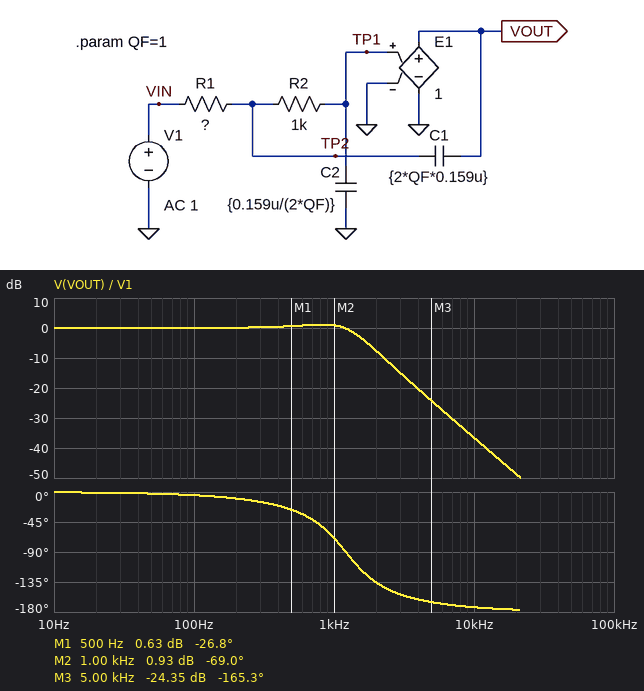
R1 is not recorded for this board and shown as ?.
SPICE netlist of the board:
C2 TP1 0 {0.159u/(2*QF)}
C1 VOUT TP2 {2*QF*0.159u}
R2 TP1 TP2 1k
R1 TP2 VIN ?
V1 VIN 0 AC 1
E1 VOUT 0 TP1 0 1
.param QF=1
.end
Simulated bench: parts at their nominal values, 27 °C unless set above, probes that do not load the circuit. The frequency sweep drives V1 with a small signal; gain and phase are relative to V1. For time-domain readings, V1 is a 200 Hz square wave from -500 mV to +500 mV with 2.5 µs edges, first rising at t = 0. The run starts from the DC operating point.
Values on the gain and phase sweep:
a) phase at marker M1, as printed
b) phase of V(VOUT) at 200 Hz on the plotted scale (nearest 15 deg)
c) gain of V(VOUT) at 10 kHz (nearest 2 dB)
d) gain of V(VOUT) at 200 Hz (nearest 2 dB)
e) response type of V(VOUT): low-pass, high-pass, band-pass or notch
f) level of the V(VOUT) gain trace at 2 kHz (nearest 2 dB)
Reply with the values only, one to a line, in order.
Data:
-26.8 deg
-15 deg
-36 dB
0 dB
low-pass
-8 dB
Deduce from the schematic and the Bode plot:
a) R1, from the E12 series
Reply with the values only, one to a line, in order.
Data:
680 Ω
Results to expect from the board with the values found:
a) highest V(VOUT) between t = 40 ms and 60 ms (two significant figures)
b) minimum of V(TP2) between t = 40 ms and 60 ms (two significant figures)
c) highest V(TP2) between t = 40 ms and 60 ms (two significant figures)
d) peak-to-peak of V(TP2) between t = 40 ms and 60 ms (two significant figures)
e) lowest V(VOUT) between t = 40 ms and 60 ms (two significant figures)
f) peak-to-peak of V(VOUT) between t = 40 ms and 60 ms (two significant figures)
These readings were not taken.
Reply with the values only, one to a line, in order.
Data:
660 mV
-700 mV
700 mV
1.4 V
-660 mV
1.3 V
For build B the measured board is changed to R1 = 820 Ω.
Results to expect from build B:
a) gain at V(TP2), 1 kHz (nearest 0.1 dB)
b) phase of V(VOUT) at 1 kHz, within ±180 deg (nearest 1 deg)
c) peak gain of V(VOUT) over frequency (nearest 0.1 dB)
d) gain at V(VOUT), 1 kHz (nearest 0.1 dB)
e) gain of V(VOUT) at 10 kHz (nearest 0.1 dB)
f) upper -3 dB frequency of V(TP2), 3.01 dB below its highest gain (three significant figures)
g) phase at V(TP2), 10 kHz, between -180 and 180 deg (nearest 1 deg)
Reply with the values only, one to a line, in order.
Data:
1.6 dB
-79 deg
1.2 dB
0.7 dB
-38.2 dB
1.39 kHz
-95 deg
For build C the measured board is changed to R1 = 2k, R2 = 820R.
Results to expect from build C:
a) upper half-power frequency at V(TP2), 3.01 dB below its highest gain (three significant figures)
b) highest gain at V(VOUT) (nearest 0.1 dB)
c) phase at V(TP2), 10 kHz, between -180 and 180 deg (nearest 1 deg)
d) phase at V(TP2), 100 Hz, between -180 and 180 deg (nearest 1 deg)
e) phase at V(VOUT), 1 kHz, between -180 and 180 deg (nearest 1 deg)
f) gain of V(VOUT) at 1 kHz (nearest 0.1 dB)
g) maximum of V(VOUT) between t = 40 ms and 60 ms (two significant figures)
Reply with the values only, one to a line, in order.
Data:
924 Hz
0.7 dB
-99 deg
-6 deg
-114 deg
-3.8 dB
630 mV
